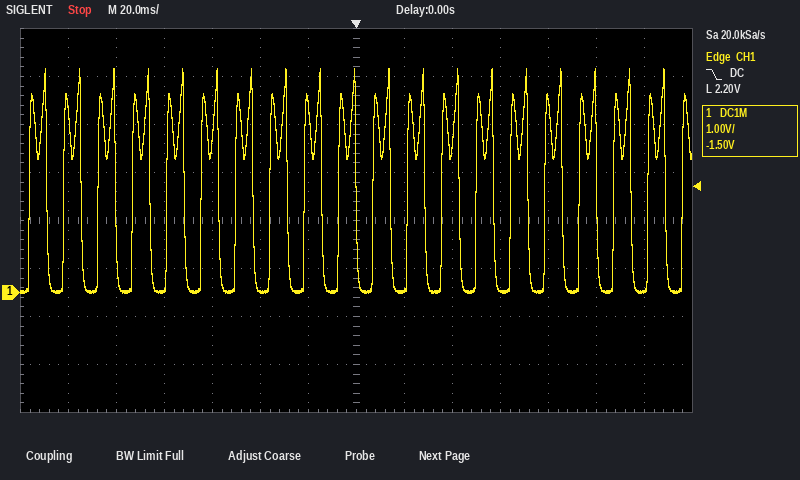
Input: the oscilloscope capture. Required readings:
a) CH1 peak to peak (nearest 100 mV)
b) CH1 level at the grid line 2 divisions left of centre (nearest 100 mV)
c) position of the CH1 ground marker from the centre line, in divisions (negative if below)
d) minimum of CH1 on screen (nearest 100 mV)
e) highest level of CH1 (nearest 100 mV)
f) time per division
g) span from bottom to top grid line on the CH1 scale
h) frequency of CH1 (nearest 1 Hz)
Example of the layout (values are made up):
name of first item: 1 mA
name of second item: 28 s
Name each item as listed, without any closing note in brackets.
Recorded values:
CH1 peak to peak: 4.7 V
CH1 level at the grid line 2 divisions left of centre: 0.0 V
position of the CH1 ground marker from the centre line, in divisions: -1.5 div
minimum of CH1 on screen: 0.0 V
highest level of CH1: 4.7 V
time per division: 20 ms
span from bottom to top grid line on the CH1 scale: 8 V
frequency of CH1: 70 Hz
